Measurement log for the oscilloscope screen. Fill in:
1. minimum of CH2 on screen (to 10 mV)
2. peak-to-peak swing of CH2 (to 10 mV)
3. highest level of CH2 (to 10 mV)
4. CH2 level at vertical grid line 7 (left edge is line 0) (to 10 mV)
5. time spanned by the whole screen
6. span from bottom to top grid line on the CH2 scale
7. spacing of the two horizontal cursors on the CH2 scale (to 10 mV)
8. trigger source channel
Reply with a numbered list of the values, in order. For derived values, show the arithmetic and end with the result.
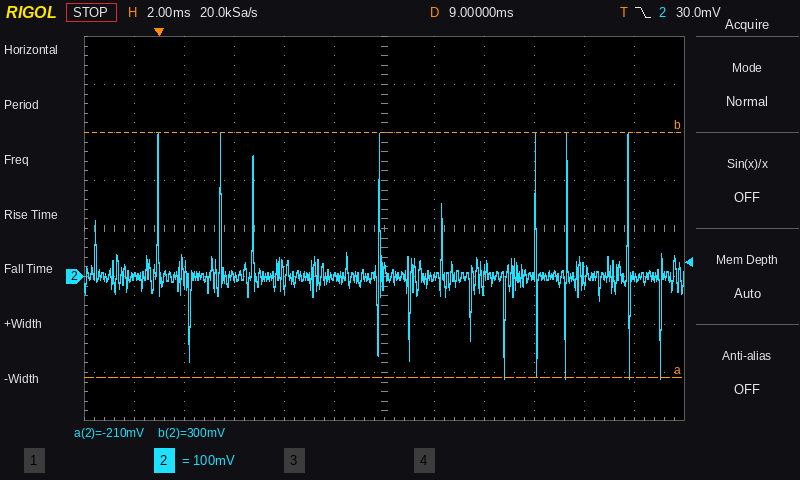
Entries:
1. -210 mV
2. 300 mV − (-210 mV) = 510 mV
3. 300 mV
4. 0 mV
5. 24 ms
6. 800 mV
7. 510 mV
8. CH2
